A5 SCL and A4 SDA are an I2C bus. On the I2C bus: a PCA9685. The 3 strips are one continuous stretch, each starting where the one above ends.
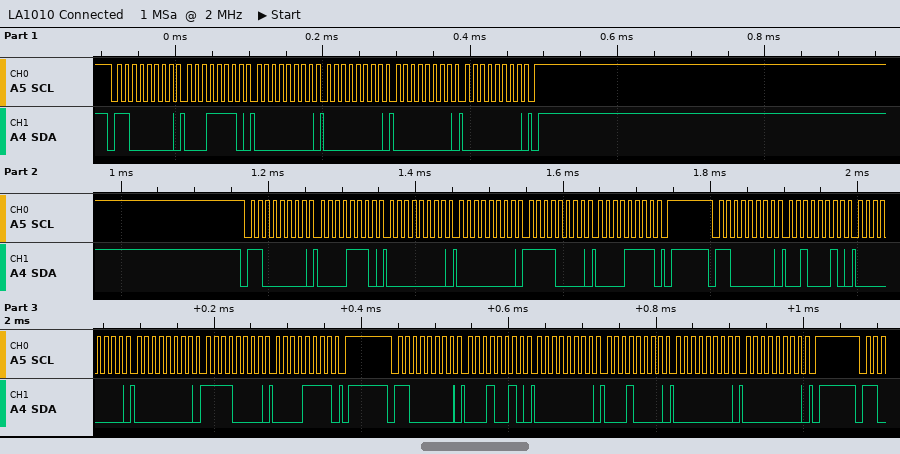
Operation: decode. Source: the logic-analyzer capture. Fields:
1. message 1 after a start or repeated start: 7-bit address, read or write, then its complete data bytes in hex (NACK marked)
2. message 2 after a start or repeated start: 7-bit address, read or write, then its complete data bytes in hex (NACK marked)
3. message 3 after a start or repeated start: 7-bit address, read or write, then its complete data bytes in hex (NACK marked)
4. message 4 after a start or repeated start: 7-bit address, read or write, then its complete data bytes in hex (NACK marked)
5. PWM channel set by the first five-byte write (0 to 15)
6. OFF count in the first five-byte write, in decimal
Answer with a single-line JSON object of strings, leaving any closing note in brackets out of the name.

{"message 1 after a start or repeated start: 7-bit address, read or write, then its complete data bytes in hex": "0x60 write: 1E 00 00 00 00", "message 2 after a start or repeated start: 7-bit address, read or write, then its complete data bytes in hex": "0x60 write: 0E 00 00 F0 0F", "message 3 after a start or repeated start: 7-bit address, read or write, then its complete data bytes in hex": "0x60 write: 22 00 00 F0 0F", "message 4 after a start or repeated start: 7-bit address, read or write, then its complete data bytes in hex": "0x60 write: 12 00 10 00 00", "PWM channel set by the first five-byte write": "6", "OFF count in the first five-byte write, in decimal": "0"}
